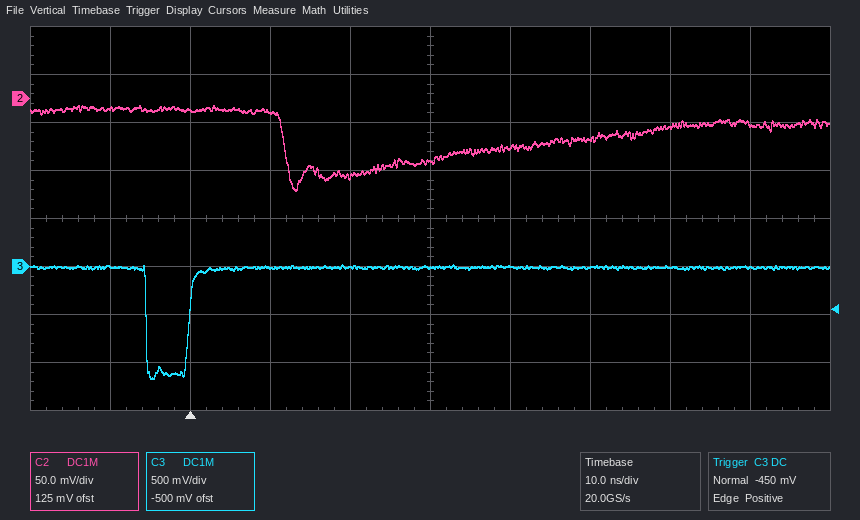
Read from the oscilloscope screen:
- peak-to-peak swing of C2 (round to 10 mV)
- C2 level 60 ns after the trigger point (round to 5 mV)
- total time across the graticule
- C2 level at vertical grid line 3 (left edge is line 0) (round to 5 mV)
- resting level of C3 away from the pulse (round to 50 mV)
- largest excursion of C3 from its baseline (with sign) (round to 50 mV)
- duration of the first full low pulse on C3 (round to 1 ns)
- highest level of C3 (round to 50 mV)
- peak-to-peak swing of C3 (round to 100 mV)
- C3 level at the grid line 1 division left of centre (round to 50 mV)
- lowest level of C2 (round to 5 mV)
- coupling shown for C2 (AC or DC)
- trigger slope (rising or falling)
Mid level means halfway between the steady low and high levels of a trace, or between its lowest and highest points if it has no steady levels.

90 mV
-30 mV
100 ns
-15 mV
0 mV
-1.15 V
5 ns
0 mV
1.20 V
0 mV
-95 mV
DC
rising
